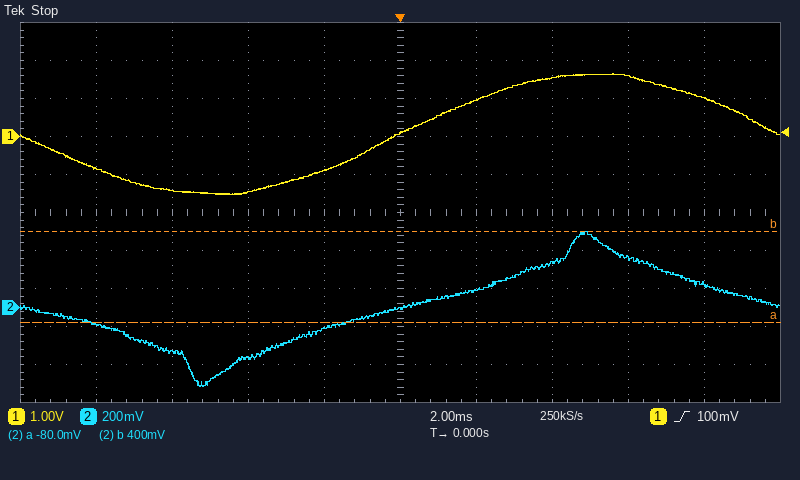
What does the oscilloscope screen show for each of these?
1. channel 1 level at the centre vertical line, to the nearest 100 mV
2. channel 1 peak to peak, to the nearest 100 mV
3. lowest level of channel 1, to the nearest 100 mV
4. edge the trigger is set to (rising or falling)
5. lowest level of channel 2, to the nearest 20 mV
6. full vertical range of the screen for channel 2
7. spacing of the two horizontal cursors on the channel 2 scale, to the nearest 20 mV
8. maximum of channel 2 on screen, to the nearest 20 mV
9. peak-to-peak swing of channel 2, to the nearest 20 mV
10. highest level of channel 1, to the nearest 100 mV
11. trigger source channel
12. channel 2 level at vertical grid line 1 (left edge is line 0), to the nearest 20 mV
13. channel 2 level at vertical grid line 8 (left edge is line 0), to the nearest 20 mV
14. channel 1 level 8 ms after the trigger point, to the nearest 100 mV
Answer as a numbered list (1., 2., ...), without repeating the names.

1. 100 mV
2. 3.2 V
3. -1.5 V
4. rising
5. -420 mV
6. 2 V
7. 480 mV
8. 400 mV
9. 820 mV
10. 1.7 V
11. channel 1
12. -80 mV
13. 260 mV
14. 1.0 V
